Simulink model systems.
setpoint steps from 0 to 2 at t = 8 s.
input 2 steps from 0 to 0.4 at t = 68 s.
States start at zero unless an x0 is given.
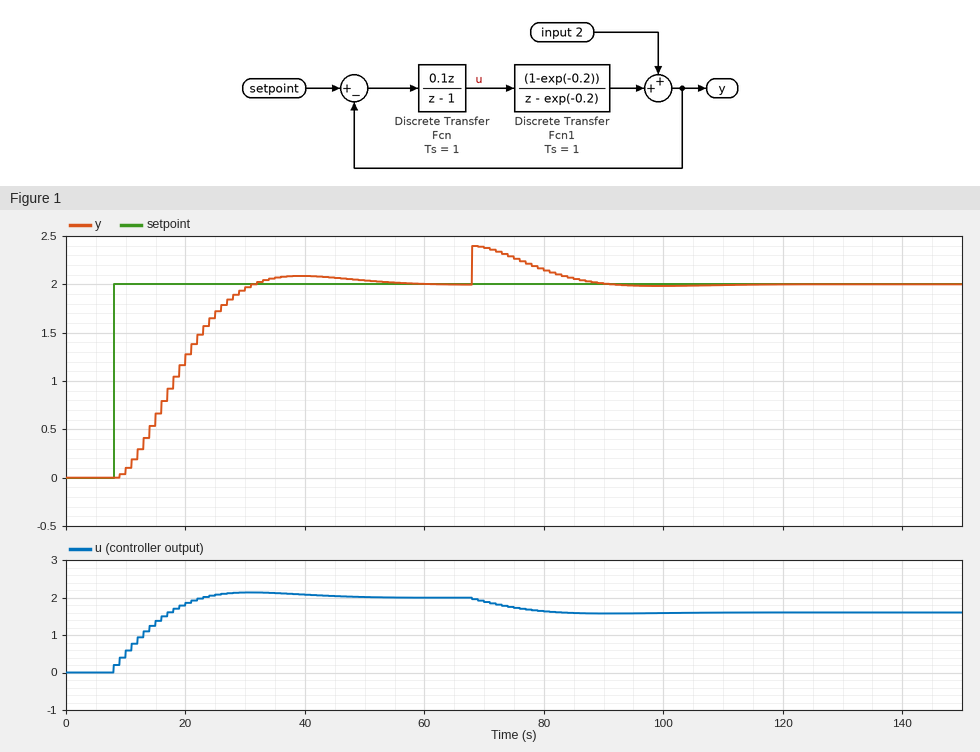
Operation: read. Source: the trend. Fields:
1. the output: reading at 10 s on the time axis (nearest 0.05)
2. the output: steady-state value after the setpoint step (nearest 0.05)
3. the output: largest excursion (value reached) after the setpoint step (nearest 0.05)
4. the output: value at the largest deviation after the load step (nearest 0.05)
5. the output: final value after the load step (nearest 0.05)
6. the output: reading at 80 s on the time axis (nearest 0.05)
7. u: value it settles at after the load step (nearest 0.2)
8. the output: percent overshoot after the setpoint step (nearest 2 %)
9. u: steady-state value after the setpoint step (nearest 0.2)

0.10
2.00
2.10
2.40
2.00
2.15
1.6
4 %
2.0
